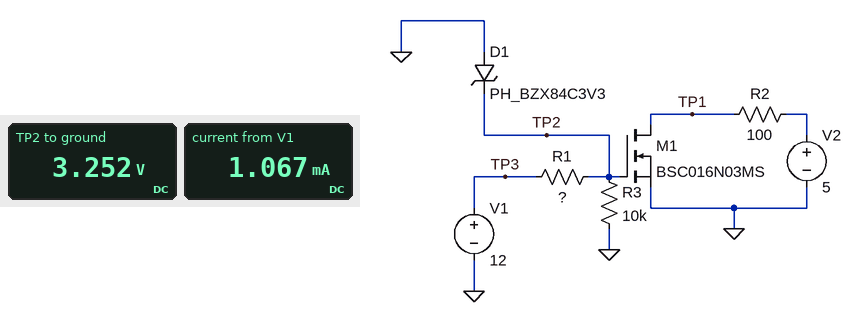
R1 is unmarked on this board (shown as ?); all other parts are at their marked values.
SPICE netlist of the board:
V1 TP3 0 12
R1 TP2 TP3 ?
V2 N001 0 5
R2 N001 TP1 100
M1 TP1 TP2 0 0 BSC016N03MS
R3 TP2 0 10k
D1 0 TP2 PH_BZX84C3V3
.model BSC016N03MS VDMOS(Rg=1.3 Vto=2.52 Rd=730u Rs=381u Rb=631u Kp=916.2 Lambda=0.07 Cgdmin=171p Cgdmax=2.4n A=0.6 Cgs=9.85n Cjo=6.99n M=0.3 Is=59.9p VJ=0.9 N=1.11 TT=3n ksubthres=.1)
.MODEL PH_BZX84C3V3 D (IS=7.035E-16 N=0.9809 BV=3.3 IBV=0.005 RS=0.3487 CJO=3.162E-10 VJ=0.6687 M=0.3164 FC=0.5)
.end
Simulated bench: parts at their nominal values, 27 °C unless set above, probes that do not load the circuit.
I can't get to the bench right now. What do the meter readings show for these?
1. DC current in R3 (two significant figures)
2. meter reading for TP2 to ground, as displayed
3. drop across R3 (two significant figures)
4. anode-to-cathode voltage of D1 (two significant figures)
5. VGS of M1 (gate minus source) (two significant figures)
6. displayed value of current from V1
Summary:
330 µA
3.252 V
3.3 V
-3.3 V
3.3 V
1.067 mA
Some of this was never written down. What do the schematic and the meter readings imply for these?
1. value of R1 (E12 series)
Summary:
8.2 kΩ
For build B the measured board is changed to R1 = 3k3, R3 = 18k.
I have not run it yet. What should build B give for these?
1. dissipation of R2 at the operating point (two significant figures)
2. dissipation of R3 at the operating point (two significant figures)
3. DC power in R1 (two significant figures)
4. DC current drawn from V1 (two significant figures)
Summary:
250 mW
600 µW
23 mW
2.6 mA
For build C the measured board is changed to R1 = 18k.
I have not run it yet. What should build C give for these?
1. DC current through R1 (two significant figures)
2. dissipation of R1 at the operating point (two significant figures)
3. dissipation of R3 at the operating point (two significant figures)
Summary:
490 µA
4.3 mW
1.0 mW
